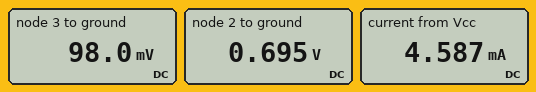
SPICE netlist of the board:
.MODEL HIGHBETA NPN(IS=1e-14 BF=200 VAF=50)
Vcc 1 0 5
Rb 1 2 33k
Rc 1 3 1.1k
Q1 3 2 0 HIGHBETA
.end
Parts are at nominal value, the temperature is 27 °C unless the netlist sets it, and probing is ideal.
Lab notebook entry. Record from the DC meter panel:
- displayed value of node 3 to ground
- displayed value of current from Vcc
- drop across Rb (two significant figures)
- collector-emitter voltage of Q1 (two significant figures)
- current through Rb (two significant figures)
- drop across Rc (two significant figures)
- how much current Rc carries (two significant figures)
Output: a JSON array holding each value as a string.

["98.0 mV", "4.587 mA", "4.3 V", "98 mV", "130 µA", "4.9 V", "4.5 mA"]
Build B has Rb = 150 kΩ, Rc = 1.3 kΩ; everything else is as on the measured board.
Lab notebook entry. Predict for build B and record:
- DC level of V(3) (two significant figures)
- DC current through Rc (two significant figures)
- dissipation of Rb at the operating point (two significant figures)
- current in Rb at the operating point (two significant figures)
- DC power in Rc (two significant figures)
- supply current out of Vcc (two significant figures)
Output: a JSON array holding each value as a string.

["150 mV", "3.7 mA", "120 µW", "29 µA", "18 mW", "3.8 mA"]
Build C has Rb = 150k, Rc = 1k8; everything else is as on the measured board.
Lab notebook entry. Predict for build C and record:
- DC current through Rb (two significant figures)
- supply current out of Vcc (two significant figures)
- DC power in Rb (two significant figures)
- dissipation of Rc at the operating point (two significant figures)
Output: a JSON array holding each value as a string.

["29 µA", "2.7 mA", "120 µW", "13 mW"]
